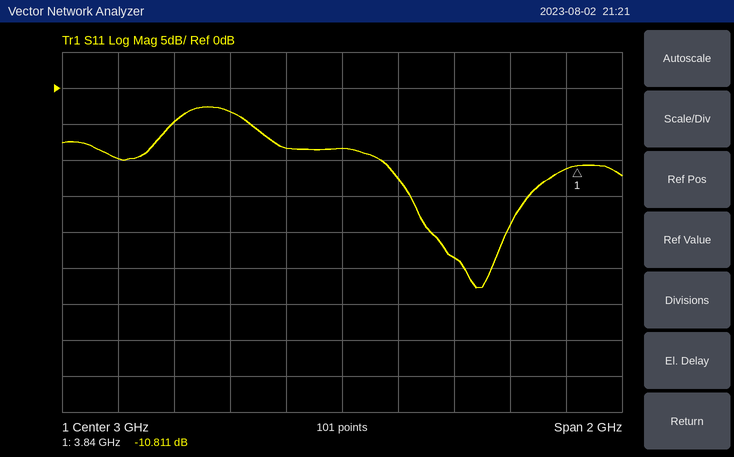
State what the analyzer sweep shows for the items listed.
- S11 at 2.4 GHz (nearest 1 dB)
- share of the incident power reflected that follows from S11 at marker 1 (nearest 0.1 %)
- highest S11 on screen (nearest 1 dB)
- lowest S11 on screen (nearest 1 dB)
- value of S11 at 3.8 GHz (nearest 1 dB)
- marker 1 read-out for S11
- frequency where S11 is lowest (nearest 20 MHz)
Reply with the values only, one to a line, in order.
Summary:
-5 dB
8.3 %
-3 dB
-28 dB
-11 dB
-10.811 dB
3.48 GHz
